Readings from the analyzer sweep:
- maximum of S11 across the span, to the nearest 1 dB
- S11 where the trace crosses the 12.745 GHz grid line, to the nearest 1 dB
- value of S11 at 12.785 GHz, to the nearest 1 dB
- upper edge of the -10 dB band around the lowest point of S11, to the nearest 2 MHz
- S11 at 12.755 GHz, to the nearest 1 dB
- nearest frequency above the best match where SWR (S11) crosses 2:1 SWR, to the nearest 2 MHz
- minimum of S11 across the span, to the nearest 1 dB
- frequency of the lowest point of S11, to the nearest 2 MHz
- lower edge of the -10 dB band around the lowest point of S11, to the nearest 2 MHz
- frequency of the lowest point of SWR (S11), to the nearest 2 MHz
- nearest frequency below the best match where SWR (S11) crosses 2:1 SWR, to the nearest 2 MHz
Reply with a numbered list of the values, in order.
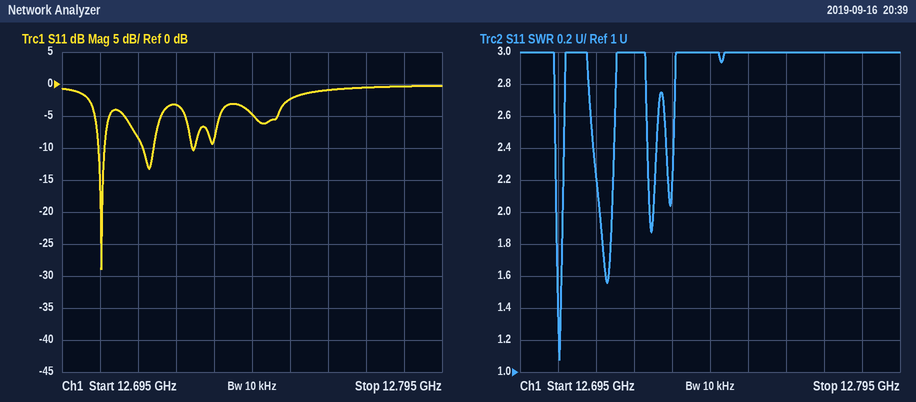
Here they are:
1. 0 dB
2. -5 dB
3. 0 dB
4. 12.706 GHz
5. -2 dB
6. 12.706 GHz
7. -29 dB
8. 12.706 GHz
9. 12.704 GHz
10. 12.706 GHz
11. 12.704 GHz
